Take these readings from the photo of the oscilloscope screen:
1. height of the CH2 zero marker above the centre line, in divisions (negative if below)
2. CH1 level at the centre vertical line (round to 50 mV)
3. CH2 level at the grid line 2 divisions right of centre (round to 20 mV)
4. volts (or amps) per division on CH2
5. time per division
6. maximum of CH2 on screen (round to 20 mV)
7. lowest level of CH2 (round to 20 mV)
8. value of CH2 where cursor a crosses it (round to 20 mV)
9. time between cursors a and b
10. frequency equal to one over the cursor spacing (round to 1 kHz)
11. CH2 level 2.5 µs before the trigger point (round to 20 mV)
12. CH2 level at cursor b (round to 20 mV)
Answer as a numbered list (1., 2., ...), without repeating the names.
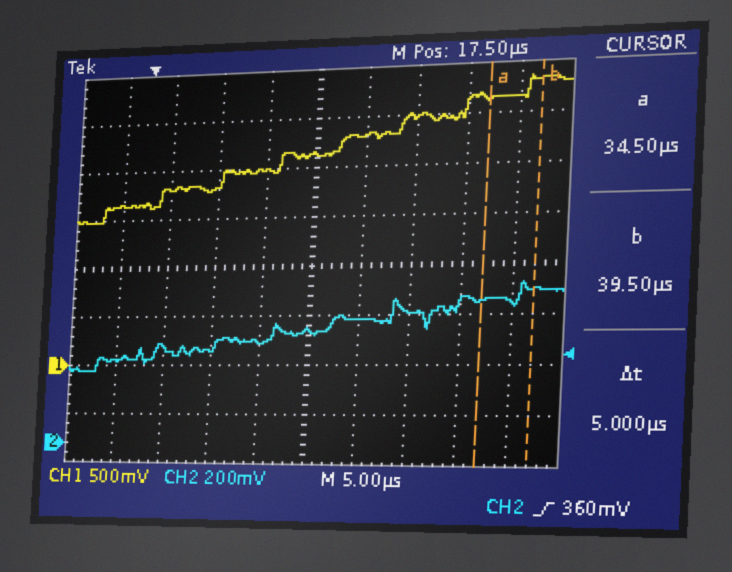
1. -3.6 div
2. 2.15 V
3. 540 mV
4. 200 mV
5. 5 µs
6. 640 mV
7. 300 mV
8. 580 mV
9. 5 µs
10. 200 kHz
11. 340 mV
12. 620 mV
